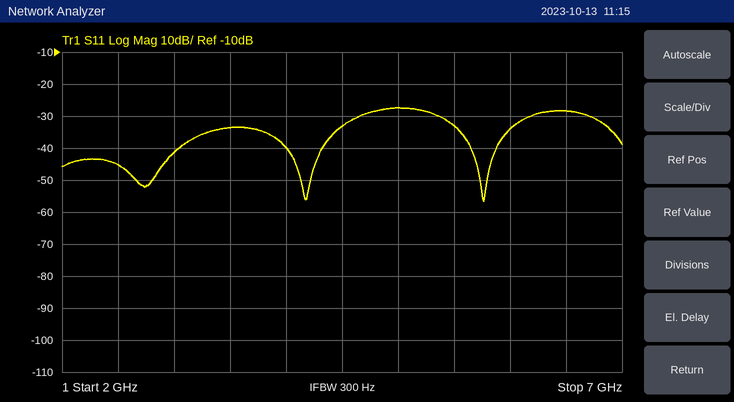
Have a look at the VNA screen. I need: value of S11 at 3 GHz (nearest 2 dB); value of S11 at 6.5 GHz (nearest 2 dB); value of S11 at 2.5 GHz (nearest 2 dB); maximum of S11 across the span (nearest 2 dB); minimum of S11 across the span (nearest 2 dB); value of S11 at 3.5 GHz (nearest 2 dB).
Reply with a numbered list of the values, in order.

1. -42 dB
2. -28 dB
3. -46 dB
4. -28 dB
5. -56 dB
6. -34 dB
